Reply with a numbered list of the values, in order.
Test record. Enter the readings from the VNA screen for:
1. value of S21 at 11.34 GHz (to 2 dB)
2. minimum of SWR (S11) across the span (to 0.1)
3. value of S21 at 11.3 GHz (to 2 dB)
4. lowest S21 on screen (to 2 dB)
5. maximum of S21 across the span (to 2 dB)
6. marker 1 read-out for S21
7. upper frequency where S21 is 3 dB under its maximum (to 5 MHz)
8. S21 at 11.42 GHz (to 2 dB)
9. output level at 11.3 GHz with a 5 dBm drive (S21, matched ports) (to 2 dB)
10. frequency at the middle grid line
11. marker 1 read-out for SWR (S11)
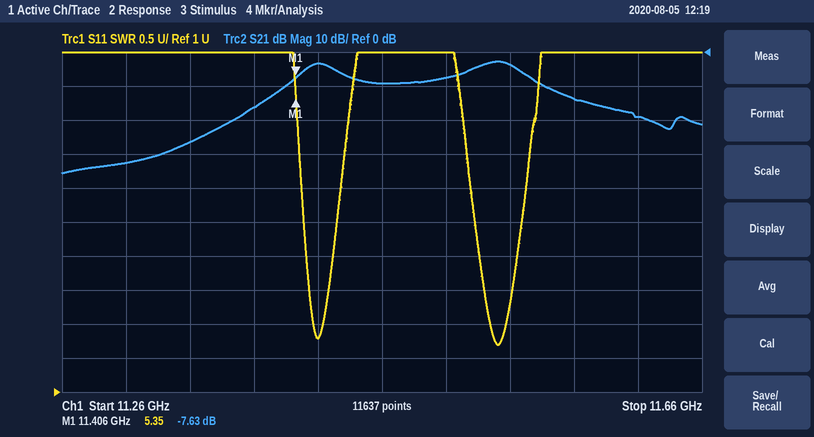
1. -26 dB
2. 1.7
3. -32 dB
4. -36 dB
5. -2 dB
6. -7.63 dB
7. 11.545 GHz
8. -4 dB
9. -28 dBm
10. 11.46 GHz
11. 5.35
